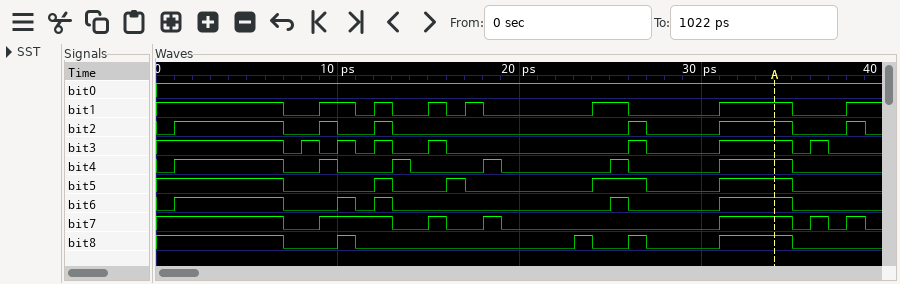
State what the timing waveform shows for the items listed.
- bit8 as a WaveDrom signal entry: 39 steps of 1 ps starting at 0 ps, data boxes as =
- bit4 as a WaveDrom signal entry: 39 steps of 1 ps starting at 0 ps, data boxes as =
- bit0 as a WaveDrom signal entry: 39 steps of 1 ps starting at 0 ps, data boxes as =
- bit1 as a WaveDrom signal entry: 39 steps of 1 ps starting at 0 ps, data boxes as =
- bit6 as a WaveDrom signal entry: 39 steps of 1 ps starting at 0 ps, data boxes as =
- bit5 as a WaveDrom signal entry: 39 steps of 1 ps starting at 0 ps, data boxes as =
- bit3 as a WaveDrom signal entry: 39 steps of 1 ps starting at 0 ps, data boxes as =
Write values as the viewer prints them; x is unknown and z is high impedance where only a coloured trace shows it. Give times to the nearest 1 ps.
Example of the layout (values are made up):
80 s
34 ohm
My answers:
{name: 'bit8', wave: '1......0..10...........10.10...1...0...'}
{name: 'bit4', wave: '01.....0.10..10...10.....10....1...0...'}
{name: 'bit0', wave: '1......................................'}
{name: 'bit1', wave: '1......0.1.010.1010.....1.0....1...0..1'}
{name: 'bit6', wave: '01.....0..1010...........10....1...0...'}
{name: 'bit5', wave: '1......0....10..10......1..0...1...0...'}
{name: 'bit3', wave: '1......0101010.10.........10...1...010.'}
